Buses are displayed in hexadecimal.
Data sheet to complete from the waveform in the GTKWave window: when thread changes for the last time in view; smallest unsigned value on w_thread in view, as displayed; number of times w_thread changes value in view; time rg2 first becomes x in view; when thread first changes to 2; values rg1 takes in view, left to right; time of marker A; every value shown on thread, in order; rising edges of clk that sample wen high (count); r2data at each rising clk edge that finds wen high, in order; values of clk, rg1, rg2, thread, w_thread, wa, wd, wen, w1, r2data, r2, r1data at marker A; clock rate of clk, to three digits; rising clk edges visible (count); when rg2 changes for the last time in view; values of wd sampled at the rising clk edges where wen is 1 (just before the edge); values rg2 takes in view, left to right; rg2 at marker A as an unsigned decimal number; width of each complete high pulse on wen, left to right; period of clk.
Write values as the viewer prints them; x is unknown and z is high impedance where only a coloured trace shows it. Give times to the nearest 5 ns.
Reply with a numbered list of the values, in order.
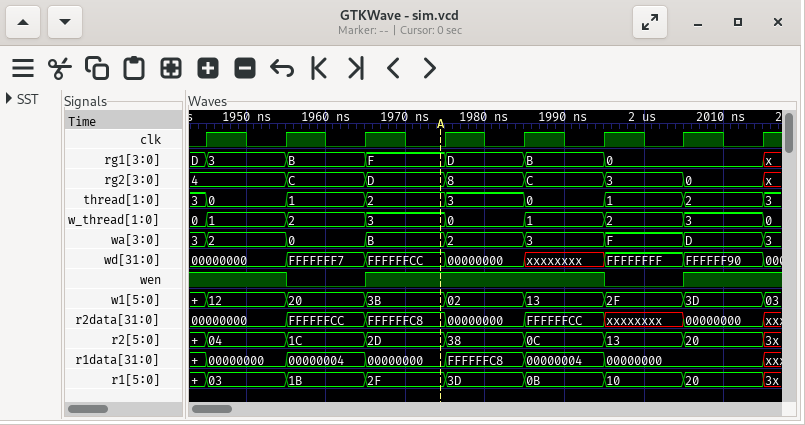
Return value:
1. 2015 ns
2. 0
3. 8
4. 2015 ns
5. 1965 ns
6. D, 3, B, F, D, B, 0, x
7. 1975 ns
8. 3, 0, 1, 2, 3, 0, 1, 2, 3
9. 6
10. 00000000, 00000000, FFFFFFC8, 00000000, FFFFFFCC, 00000000
11. clk=0, rg1=F, rg2=D, thread=2, w_thread=3, wa=B, wd=FFFFFFCC, wen=1, w1=3B, r2data=FFFFFFC8, r2=2D, r1data=00000000
12. 100 MHz
13. 8
14. 2015 ns
15. 00000000, 00000000, FFFFFFCC, 00000000, xxxxxxxx, FFFFFF90
16. 4, C, D, 8, C, 3, 0, x
17. 13
18. 30 ns
19. 10 ns
